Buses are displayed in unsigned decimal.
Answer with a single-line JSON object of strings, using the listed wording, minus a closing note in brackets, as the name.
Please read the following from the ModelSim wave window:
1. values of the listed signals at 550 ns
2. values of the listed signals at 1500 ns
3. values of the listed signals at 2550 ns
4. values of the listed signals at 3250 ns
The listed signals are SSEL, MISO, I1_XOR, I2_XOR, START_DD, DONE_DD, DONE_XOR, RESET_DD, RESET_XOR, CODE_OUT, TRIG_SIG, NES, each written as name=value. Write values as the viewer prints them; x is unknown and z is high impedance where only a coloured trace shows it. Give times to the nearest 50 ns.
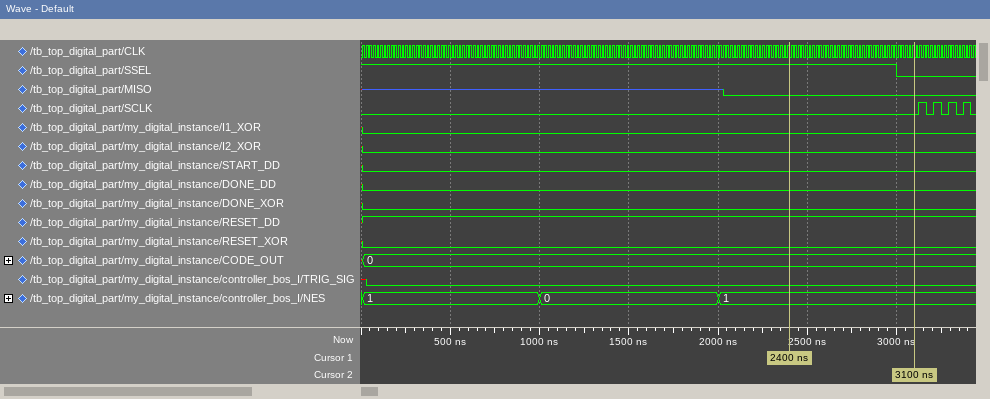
{"values of the listed signals at 550 ns": "SSEL=1, MISO=z, I1_XOR=0, I2_XOR=0, START_DD=0, DONE_DD=0, DONE_XOR=0, RESET_DD=1, RESET_XOR=0, CODE_OUT=0, TRIG_SIG=0, NES=1", "values of the listed signals at 1500 ns": "SSEL=1, MISO=z, I1_XOR=0, I2_XOR=0, START_DD=0, DONE_DD=0, DONE_XOR=0, RESET_DD=1, RESET_XOR=0, CODE_OUT=0, TRIG_SIG=0, NES=0", "values of the listed signals at 2550 ns": "SSEL=1, MISO=0, I1_XOR=0, I2_XOR=0, START_DD=0, DONE_DD=0, DONE_XOR=0, RESET_DD=1, RESET_XOR=0, CODE_OUT=0, TRIG_SIG=0, NES=1", "values of the listed signals at 3250 ns": "SSEL=0, MISO=0, I1_XOR=0, I2_XOR=0, START_DD=0, DONE_DD=0, DONE_XOR=0, RESET_DD=1, RESET_XOR=0, CODE_OUT=0, TRIG_SIG=0, NES=1"}
